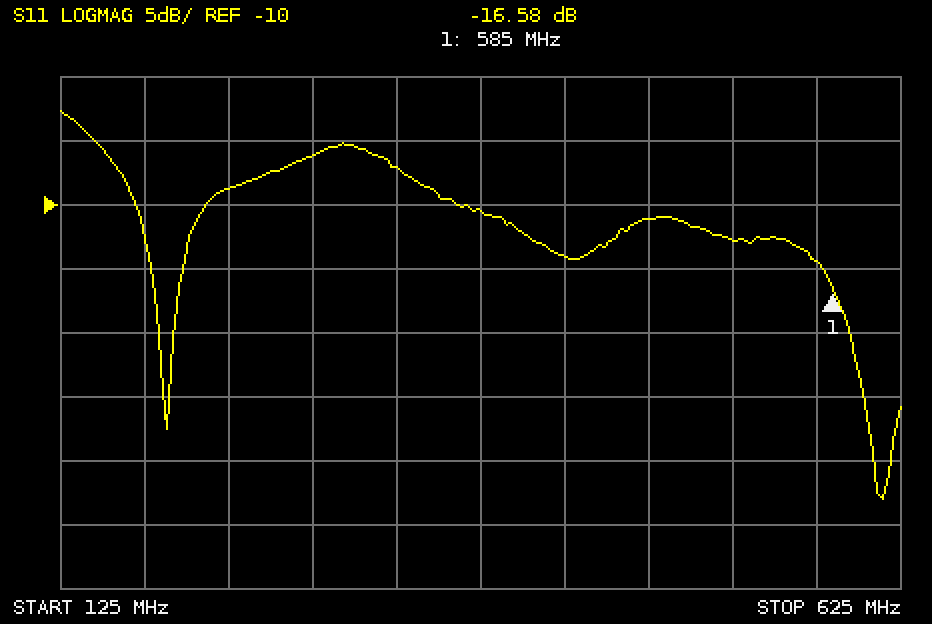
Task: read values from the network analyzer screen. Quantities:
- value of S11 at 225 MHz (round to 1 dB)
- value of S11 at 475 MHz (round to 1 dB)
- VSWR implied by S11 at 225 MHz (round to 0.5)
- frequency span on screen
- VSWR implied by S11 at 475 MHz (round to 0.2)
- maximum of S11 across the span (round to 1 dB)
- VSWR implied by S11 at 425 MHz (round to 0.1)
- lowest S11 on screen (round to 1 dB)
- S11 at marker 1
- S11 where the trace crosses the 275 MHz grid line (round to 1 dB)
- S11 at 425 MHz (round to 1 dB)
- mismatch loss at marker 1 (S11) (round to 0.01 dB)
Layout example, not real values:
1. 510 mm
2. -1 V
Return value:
1. -9 dB
2. -11 dB
3. 2.0
4. 500 MHz
5. 1.8
6. -3 dB
7. 1.5
8. -33 dB
9. -16.58 dB
10. -6 dB
11. -14 dB
12. 0.10 dB
